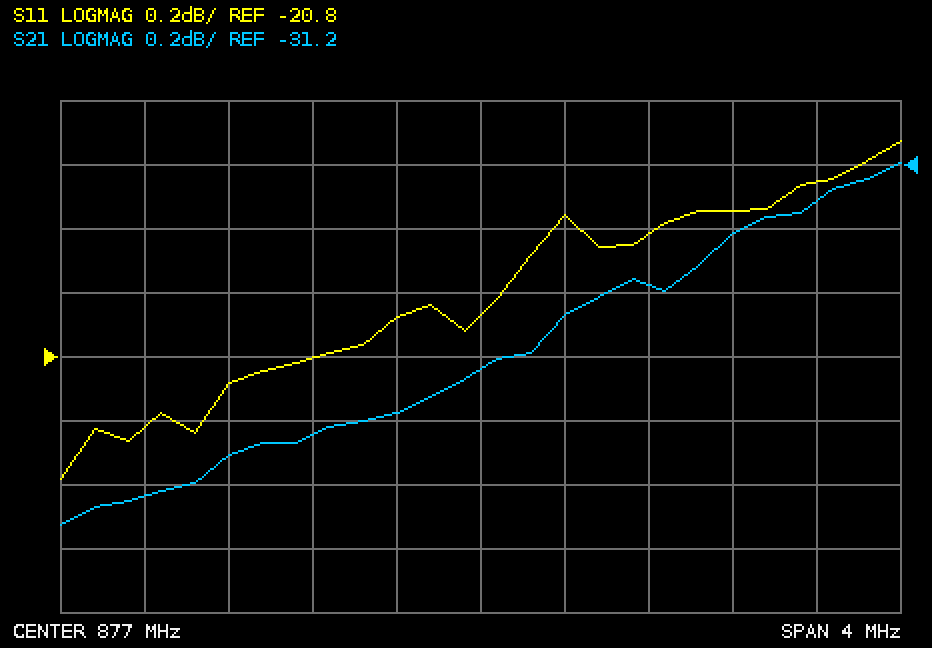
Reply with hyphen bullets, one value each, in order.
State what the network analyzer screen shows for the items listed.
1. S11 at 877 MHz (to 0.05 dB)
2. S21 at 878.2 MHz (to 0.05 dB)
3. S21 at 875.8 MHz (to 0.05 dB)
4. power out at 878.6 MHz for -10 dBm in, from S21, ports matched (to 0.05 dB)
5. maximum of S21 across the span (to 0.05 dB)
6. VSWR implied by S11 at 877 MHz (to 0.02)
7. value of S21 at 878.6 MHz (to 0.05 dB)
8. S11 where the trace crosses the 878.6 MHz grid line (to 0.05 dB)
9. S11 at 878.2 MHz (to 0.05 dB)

- -20.65 dB
- -31.40 dB
- -32.10 dB
- -41.30 dBm
- -31.20 dB
- 1.20
- -31.30 dB
- -20.25 dB
- -20.35 dB
